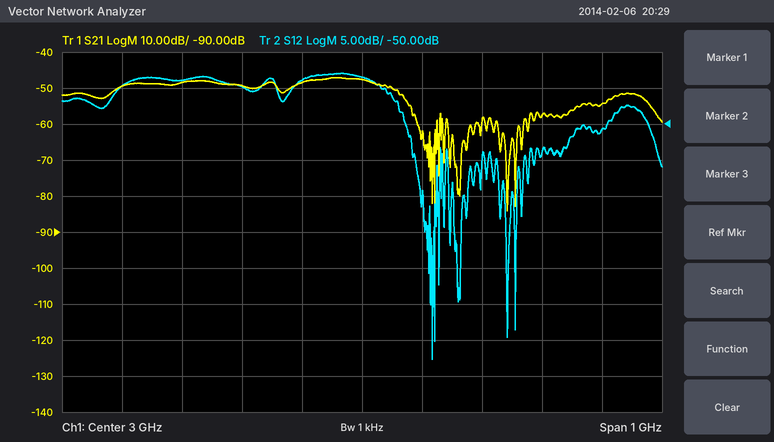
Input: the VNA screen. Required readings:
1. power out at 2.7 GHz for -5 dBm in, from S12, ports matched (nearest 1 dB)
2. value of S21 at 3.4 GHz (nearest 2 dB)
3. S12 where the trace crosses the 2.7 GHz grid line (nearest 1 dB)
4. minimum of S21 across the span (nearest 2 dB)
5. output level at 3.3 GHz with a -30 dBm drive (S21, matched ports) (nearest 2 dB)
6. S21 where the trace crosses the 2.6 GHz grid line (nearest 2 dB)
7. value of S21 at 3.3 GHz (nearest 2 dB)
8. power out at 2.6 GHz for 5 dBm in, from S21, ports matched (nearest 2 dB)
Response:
-49 dBm
-54 dB
-44 dB
-84 dB
-88 dBm
-50 dB
-58 dB
-44 dBm
